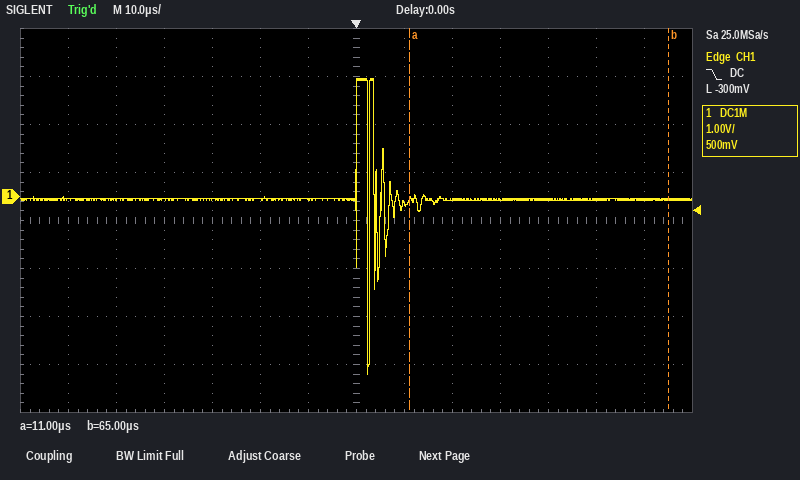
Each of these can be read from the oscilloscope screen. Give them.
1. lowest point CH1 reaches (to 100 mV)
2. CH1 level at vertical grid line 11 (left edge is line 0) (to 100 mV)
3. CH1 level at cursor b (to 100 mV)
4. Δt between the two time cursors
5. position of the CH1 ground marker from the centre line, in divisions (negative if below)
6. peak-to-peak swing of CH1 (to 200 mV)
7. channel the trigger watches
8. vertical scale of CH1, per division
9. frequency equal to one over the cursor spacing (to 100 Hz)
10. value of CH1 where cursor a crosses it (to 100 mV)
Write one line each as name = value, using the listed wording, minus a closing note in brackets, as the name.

lowest point CH1 reaches = -3.7 V
CH1 level at vertical grid line 11 (left edge is line 0) = -100 mV
CH1 level at cursor b = -100 mV
Δt between the two time cursors = 54 µs
position of the CH1 ground marker from the centre line, in divisions = +0.5 div
peak-to-peak swing of CH1 = 6.2 V
channel the trigger watches = CH1
vertical scale of CH1, per division = 1 V
frequency equal to one over the cursor spacing = 18.5 kHz
value of CH1 where cursor a crosses it = -100 mV
